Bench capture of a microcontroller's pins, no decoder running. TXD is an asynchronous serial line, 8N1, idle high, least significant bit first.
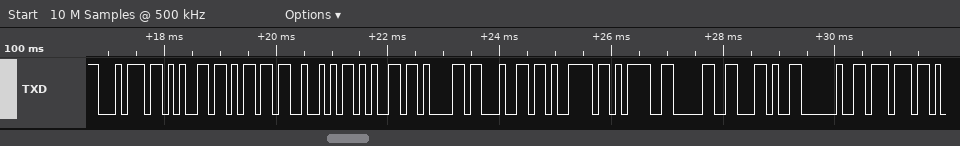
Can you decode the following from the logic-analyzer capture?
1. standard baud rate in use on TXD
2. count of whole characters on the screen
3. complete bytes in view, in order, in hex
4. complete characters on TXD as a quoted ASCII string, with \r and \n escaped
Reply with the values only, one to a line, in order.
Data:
9600 baud
13
74 65 6D 52 65 61 64 79 3D 30 2C 20 77
"temReady=0, w"
